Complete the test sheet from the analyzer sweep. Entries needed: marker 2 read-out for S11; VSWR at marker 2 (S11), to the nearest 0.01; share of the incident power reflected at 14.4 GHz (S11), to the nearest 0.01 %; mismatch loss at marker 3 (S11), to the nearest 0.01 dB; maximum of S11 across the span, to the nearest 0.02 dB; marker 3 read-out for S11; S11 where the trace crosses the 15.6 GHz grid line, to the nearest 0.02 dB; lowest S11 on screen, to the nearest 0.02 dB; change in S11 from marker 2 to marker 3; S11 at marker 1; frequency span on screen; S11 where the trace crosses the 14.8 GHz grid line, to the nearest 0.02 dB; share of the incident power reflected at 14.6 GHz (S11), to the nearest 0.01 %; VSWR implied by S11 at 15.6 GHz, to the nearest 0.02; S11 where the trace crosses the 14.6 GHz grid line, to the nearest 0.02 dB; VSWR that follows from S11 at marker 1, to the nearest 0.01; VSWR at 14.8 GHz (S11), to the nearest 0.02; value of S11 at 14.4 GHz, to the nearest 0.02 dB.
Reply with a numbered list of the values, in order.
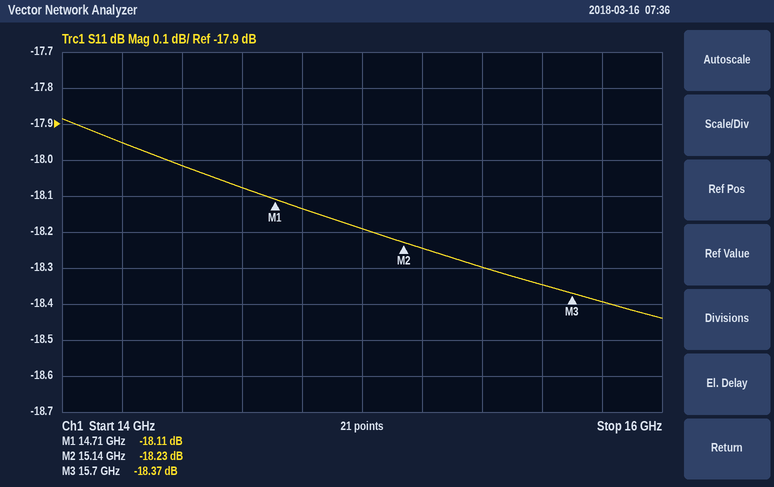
1. -18.23 dB
2. 1.28
3. 1.58 %
4. 0.06 dB
5. -17.88 dB
6. -18.37 dB
7. -18.34 dB
8. -18.44 dB
9. -0.14 dB
10. -18.11 dB
11. 2 GHz
12. -18.14 dB
13. 1.56 %
14. 1.28
15. -18.08 dB
16. 1.28
17. 1.28
18. -18.02 dB
